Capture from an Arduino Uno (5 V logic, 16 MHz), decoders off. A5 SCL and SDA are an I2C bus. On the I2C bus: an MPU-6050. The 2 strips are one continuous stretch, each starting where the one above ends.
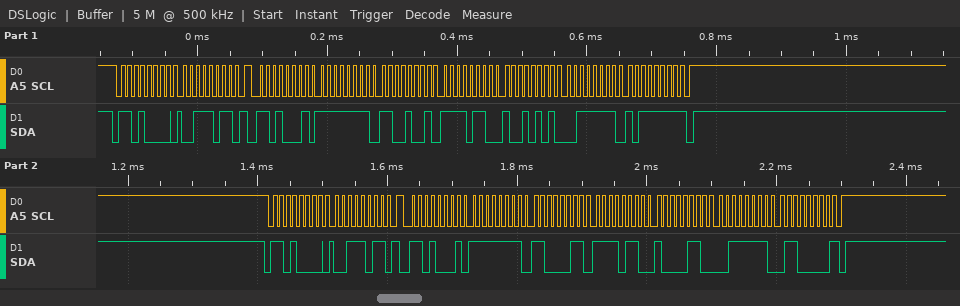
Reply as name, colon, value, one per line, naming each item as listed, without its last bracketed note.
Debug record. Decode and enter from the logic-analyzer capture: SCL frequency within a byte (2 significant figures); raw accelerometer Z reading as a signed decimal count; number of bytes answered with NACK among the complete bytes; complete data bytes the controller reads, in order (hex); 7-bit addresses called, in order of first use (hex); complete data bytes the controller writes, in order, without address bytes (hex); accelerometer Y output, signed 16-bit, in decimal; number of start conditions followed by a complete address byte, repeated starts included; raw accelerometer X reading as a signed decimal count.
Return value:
SCL frequency within a byte: 100 kHz
raw accelerometer Z reading as a signed decimal count: 16319
number of bytes answered with NACK among the complete bytes: 2
complete data bytes the controller reads, in order: FF C9 F6 95 3F BF FF C3 F6 86 3F 60
7-bit addresses called, in order of first use: 0x68
complete data bytes the controller writes, in order, without address bytes: 3B 3B
accelerometer Y output, signed 16-bit, in decimal: -2411
number of start conditions followed by a complete address byte, repeated starts included: 4
raw accelerometer X reading as a signed decimal count: -55
